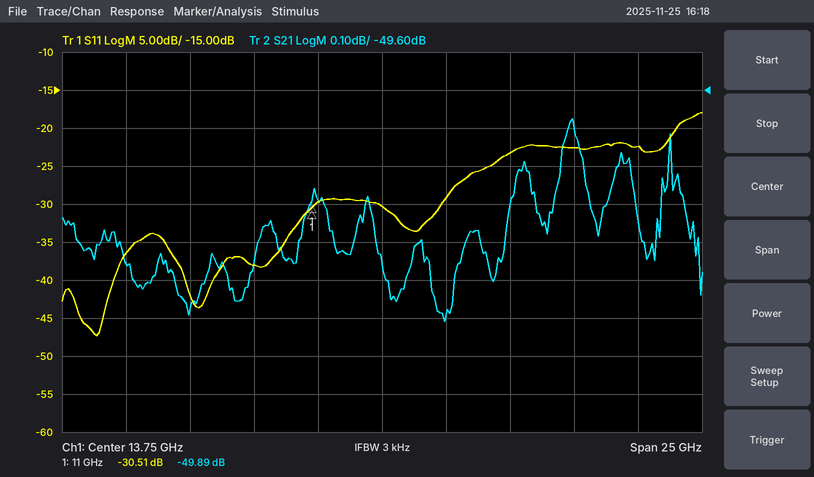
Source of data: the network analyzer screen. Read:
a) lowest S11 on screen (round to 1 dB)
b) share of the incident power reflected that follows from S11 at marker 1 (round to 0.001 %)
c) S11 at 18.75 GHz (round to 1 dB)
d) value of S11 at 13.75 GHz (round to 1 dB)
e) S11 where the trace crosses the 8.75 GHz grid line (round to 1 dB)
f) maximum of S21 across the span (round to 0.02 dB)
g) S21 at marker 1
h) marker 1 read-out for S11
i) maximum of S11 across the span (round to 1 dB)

-47 dB
0.089 %
-23 dB
-30 dB
-38 dB
-49.68 dB
-49.89 dB
-30.51 dB
-18 dB
